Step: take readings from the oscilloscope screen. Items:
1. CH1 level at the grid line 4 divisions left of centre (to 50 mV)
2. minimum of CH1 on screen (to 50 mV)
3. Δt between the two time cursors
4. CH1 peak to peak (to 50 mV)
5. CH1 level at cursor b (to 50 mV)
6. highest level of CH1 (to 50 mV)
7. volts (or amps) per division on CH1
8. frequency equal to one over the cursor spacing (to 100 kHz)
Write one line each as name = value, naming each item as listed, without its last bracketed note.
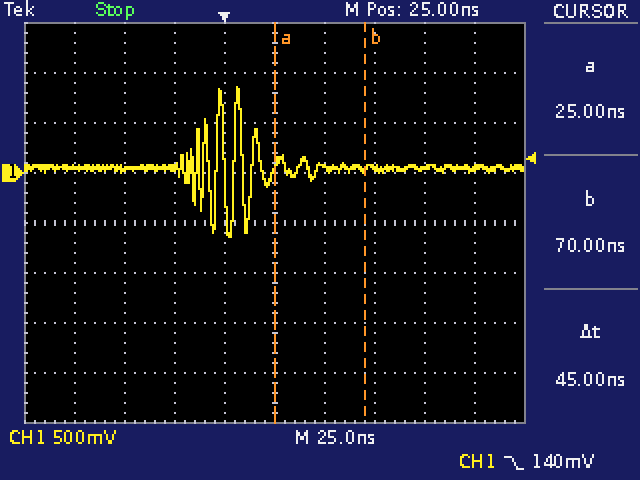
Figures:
CH1 level at the grid line 4 divisions left of centre = 50 mV
minimum of CH1 on screen = -650 mV
Δt between the two time cursors = 45 ns
CH1 peak to peak = 1.50 V
CH1 level at cursor b = 50 mV
highest level of CH1 = 850 mV
volts (or amps) per division on CH1 = 500 mV
frequency equal to one over the cursor spacing = 22.2 MHz
